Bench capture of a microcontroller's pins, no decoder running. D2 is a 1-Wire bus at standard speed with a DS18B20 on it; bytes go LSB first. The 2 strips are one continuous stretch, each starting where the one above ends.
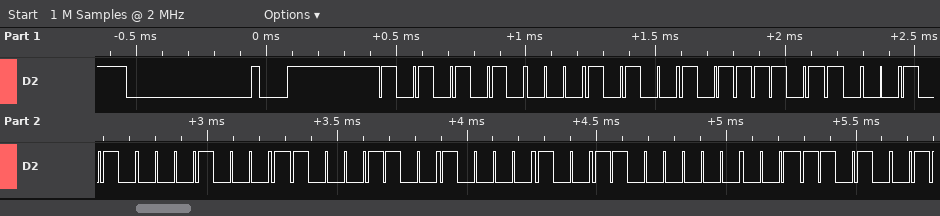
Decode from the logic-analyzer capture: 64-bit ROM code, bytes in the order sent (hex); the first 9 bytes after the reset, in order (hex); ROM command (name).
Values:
28 BD 51 88 31 21 03 5C
55 28 BD 51 88 31 21 03 5C
Match ROM
